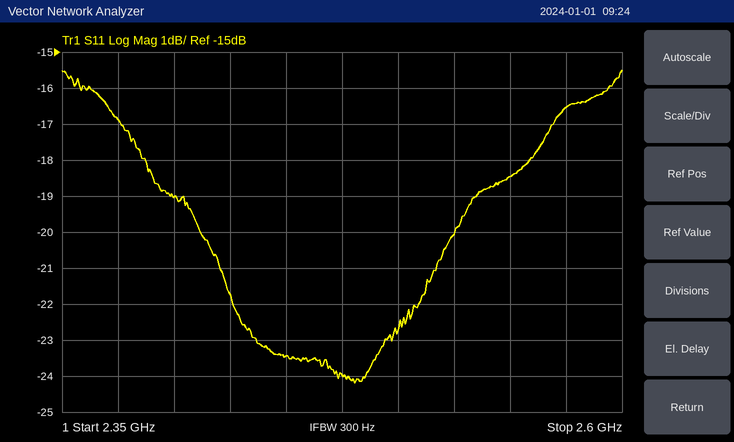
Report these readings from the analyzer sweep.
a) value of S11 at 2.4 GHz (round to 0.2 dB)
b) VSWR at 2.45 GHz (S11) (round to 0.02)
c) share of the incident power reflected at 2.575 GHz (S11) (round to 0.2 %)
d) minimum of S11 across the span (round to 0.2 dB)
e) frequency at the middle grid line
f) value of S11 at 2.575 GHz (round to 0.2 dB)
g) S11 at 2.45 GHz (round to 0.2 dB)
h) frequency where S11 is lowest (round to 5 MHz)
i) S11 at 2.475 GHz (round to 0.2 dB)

-19.0 dB
1.14
2.2 %
-24.2 dB
2.475 GHz
-16.6 dB
-23.4 dB
2.480 GHz
-24.0 dB
